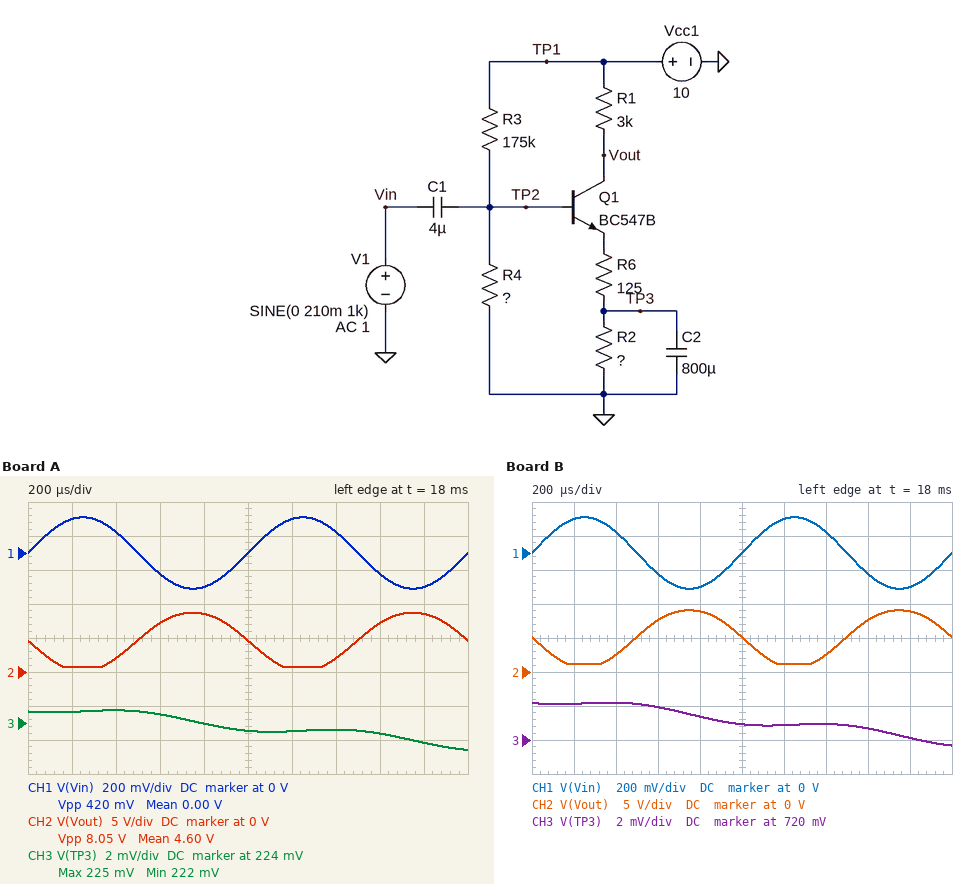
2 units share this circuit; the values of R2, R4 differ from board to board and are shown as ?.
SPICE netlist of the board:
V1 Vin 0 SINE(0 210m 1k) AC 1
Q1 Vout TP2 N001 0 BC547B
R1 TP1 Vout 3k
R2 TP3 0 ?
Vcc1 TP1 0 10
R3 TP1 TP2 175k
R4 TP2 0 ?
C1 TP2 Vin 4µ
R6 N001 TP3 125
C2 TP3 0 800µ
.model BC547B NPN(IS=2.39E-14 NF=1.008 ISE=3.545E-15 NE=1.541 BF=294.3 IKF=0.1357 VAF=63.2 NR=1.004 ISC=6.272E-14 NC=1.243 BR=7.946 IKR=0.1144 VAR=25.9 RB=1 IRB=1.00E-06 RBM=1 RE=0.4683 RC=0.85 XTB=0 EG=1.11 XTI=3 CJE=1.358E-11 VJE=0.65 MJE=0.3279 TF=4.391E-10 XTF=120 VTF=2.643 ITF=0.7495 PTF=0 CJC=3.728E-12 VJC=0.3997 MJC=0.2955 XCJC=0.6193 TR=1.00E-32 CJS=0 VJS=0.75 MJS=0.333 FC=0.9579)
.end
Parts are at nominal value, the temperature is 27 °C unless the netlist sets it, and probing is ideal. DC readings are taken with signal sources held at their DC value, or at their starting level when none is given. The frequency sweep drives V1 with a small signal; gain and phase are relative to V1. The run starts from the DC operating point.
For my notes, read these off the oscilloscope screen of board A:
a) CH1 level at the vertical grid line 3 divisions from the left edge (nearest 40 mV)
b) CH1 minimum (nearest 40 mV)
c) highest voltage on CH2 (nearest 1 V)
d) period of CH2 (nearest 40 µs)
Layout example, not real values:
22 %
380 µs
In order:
-120 mV
-200 mV
9 V
1.00 ms
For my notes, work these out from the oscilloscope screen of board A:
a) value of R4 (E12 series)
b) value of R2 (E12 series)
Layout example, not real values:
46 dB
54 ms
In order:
33 kΩ
82 Ω
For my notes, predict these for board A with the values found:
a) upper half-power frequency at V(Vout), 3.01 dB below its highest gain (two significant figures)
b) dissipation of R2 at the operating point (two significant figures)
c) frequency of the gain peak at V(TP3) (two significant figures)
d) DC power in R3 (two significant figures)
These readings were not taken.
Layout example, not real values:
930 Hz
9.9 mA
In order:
11 MHz
730 µW
2.9 Hz
430 µW
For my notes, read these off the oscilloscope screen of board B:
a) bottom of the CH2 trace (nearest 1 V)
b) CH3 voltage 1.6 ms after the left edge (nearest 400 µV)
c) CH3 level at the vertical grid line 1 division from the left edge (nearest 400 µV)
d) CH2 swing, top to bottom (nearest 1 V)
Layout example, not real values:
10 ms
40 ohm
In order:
1 V
720.8 mV
722.0 mV
8 V
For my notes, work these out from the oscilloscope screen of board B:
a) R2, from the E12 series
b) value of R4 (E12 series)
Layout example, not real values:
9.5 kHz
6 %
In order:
270 Ω
47 kΩ
